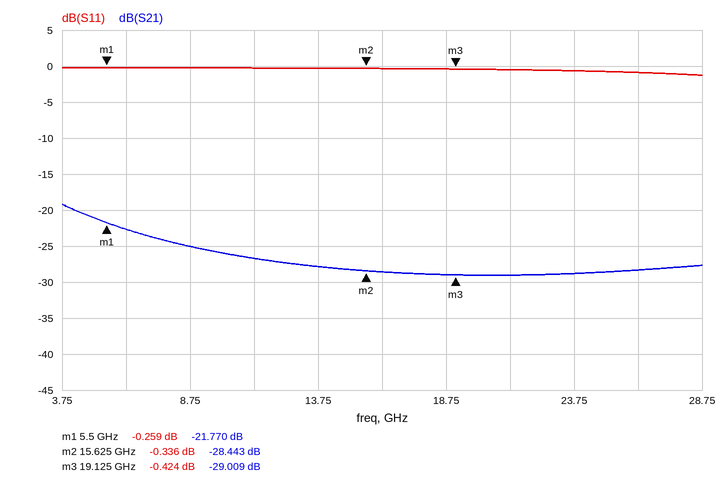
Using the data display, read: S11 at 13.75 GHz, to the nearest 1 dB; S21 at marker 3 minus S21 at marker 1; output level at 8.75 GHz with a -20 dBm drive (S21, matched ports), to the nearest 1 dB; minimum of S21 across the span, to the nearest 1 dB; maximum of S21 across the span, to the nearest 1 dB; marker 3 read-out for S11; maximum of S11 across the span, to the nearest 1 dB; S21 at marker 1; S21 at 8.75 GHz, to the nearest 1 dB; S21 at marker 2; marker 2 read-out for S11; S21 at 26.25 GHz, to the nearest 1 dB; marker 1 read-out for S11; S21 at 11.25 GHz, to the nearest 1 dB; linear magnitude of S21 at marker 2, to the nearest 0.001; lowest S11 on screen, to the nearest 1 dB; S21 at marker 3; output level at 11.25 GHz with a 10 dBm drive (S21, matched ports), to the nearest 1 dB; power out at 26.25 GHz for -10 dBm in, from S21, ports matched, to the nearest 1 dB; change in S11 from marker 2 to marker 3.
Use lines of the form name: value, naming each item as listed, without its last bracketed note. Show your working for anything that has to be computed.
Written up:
S11 at 13.75 GHz, to the nearest 1 dB: 0 dB
S21 at marker 3 minus S21 at marker 1: -29.009 − (-21.77) = -7.239 dB
output level at 8.75 GHz with a -20 dBm drive (S21, matched ports), to the nearest 1 dB: -20 dBm + (-25 dB) = -45 dBm
minimum of S21 across the span, to the nearest 1 dB: -29 dB
maximum of S21 across the span, to the nearest 1 dB: -19 dB
marker 3 read-out for S11: -0.424 dB
maximum of S11 across the span, to the nearest 1 dB: 0 dB
S21 at marker 1: -21.770 dB
S21 at 8.75 GHz, to the nearest 1 dB: -25 dB
S21 at marker 2: -28.443 dB
marker 2 read-out for S11: -0.336 dB
S21 at 26.25 GHz, to the nearest 1 dB: -28 dB
marker 1 read-out for S11: -0.259 dB
S21 at 11.25 GHz, to the nearest 1 dB: -27 dB
linear magnitude of S21 at marker 2, to the nearest 0.001: 10^(-28.443/20) ≈ 0.038
lowest S11 on screen, to the nearest 1 dB: -1 dB
S21 at marker 3: -29.009 dB
output level at 11.25 GHz with a 10 dBm drive (S21, matched ports), to the nearest 1 dB: 10 dBm + (-27 dB) = -17 dBm
power out at 26.25 GHz for -10 dBm in, from S21, ports matched, to the nearest 1 dB: -10 dBm + (-28 dB) = -38 dBm
change in S11 from marker 2 to marker 3: -0.424 − (-0.336) = -0.088 dB
